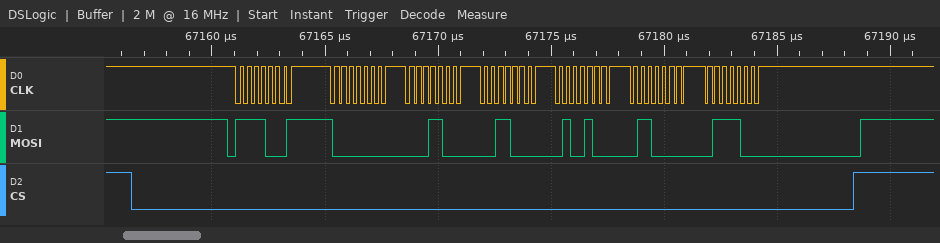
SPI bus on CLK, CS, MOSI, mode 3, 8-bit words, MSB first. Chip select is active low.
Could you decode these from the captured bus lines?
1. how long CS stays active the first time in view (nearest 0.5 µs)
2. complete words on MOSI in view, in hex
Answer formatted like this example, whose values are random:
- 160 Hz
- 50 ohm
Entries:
- 32 µs
- F1, 00, 18, 30, 48, 60, 78
